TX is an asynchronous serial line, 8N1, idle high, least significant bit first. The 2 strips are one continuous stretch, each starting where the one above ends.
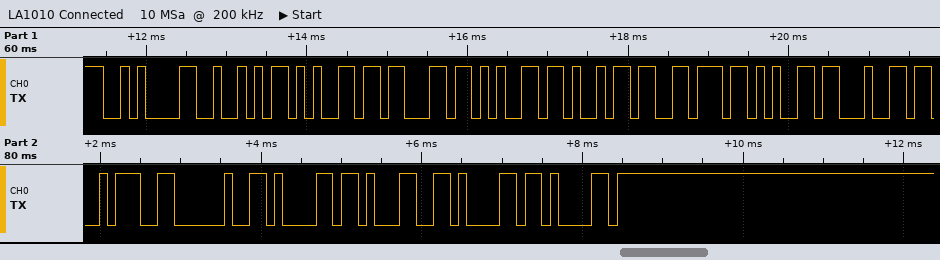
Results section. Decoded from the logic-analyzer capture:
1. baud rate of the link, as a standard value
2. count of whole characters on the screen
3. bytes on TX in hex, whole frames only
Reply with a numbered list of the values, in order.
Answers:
1. 9600 baud
2. 15
3. 0A 52 65 63 65 69 76 65 64 3A 20 61 31 61 61
